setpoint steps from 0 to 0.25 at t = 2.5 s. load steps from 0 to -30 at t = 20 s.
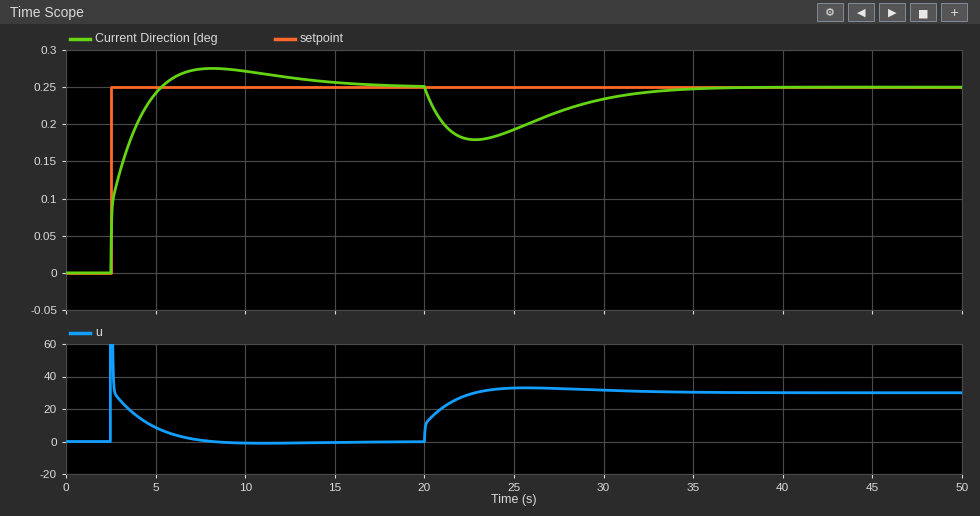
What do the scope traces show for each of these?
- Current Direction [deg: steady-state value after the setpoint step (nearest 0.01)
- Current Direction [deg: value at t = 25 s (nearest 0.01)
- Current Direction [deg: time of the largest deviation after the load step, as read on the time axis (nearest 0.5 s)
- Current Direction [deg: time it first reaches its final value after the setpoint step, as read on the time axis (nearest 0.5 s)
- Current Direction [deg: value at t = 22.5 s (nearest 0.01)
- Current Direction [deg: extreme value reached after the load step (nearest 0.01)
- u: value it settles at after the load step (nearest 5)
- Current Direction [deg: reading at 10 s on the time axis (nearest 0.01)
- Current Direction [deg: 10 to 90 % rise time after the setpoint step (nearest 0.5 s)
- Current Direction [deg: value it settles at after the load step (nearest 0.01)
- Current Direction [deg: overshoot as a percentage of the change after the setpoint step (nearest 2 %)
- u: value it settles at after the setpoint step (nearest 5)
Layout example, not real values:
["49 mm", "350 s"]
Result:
["0.25", "0.19", "23.0 s", "5.5 s", "0.18", "0.18", "30", "0.27", "2.0 s", "0.25", "10 %", "0"]
